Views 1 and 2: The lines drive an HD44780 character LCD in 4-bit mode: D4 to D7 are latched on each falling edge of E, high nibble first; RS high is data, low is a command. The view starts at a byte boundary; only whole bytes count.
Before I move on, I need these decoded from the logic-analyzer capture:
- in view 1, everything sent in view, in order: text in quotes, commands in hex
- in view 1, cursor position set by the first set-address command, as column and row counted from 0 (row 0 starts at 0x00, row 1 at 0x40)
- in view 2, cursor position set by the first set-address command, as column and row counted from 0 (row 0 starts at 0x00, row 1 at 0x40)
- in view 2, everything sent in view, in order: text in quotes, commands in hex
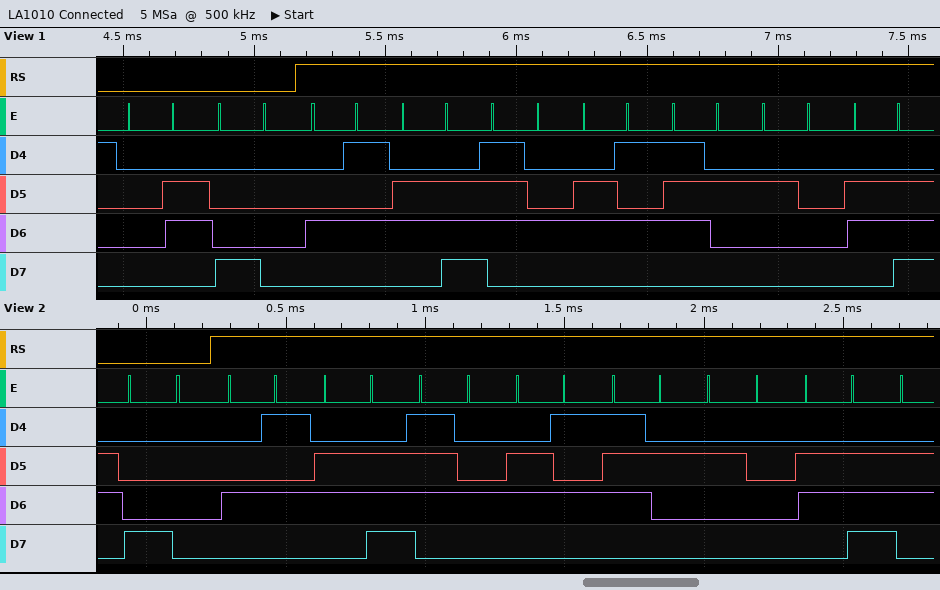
0x06 0x80 "Enter n"
column 0, row 0
column 0, row 0
0x80 "Enter n"
